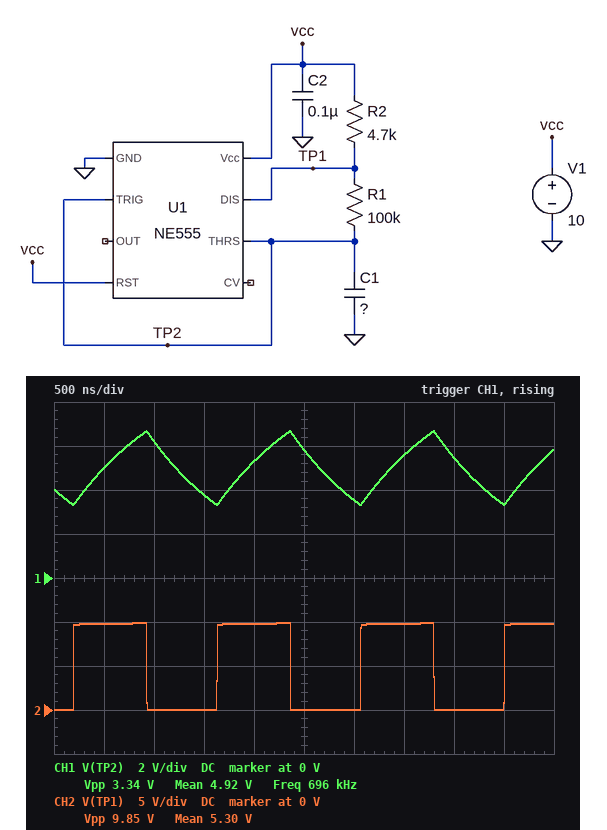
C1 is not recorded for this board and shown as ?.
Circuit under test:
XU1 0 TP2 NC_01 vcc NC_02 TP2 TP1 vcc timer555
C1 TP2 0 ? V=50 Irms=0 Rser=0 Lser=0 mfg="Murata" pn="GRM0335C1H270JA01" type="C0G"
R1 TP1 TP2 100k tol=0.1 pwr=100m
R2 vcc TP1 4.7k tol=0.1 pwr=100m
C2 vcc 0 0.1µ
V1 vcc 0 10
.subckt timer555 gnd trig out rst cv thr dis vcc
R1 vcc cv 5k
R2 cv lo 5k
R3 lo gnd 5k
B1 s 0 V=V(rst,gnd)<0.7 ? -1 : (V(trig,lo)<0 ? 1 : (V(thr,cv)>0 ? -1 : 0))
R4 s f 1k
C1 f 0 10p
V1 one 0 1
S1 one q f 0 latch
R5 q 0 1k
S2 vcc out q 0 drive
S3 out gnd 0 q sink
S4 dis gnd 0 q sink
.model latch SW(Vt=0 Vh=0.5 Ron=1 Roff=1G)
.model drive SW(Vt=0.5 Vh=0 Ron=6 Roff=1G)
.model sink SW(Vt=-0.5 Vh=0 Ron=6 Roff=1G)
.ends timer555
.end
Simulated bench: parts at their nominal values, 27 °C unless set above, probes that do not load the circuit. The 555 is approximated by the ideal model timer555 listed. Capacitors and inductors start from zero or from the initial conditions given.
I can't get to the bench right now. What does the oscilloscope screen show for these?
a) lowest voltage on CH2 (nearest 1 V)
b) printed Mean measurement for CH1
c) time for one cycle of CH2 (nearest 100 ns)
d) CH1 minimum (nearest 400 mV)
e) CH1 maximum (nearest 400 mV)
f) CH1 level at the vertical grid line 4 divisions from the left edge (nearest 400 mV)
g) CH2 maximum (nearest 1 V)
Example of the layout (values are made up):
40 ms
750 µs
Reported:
0 V
4.92 V
1.4 µs
3.2 V
6.8 V
5.2 V
10 V
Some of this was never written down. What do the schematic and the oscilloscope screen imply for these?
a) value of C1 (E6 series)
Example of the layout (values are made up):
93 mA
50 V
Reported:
10 pF
